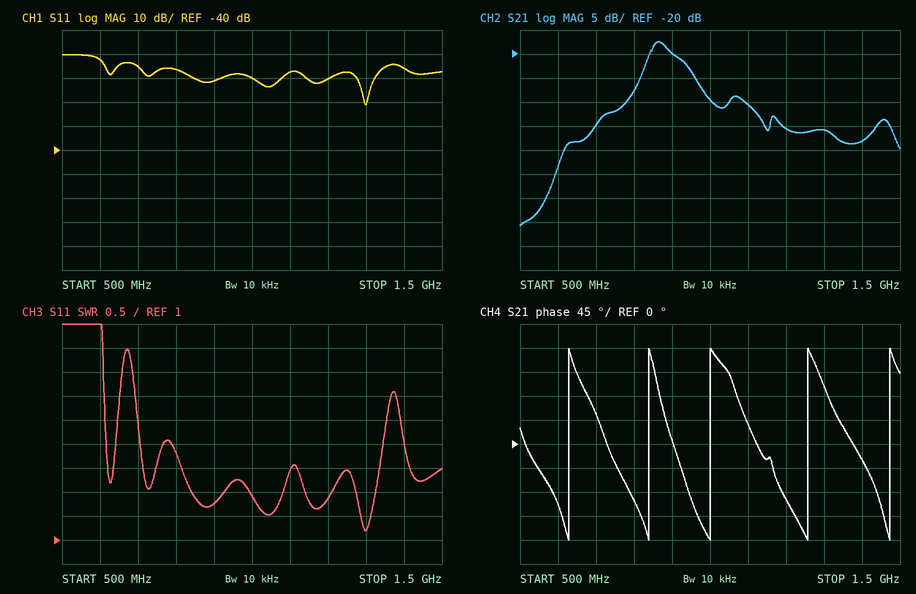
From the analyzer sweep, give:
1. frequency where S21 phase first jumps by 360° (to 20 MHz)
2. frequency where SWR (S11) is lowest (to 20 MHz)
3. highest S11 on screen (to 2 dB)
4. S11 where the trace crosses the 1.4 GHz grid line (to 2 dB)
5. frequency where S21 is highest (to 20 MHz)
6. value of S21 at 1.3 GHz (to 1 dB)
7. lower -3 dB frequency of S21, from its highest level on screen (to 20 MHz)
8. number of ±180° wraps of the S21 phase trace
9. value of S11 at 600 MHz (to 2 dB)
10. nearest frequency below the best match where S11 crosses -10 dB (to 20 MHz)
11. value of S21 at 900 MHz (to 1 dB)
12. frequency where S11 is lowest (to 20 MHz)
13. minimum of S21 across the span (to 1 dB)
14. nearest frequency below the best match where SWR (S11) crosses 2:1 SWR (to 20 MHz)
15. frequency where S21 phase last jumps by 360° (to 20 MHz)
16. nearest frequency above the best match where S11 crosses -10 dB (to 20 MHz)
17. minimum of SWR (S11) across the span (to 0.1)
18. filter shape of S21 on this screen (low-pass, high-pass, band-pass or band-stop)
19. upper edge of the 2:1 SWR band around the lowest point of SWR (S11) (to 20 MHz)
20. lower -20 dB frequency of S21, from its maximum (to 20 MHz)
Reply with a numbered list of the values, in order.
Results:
1. 620 MHz
2. 1.30 GHz
3. 0 dB
4. -6 dB
5. 860 MHz
6. -36 dB
7. 840 MHz
8. 5
9. -2 dB
10. 1.28 GHz
11. -20 dB
12. 1.30 GHz
13. -56 dB
14. 1.28 GHz
15. 1.48 GHz
16. 1.32 GHz
17. 1.2
18. band-pass
19. 1.32 GHz
20. 680 MHz
